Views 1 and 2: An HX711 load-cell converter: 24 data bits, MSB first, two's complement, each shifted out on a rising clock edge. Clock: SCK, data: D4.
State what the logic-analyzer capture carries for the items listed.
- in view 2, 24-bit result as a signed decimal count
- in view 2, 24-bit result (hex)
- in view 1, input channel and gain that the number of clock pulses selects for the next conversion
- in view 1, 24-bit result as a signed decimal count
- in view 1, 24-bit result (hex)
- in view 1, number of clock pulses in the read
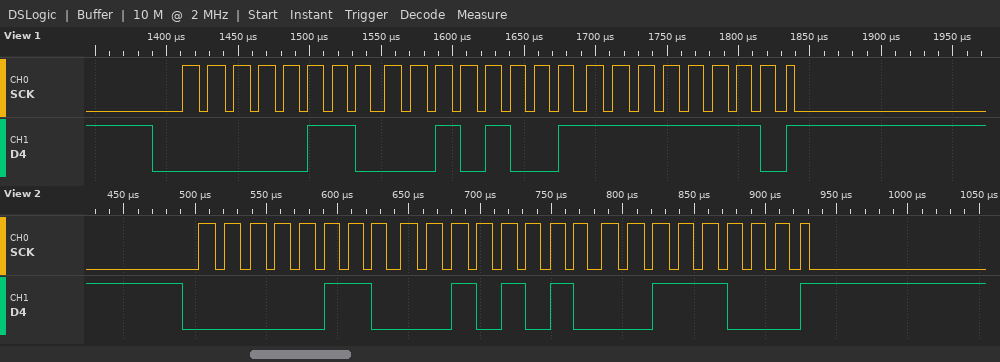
404024
0x062A38
channel A, gain 128
403966
0x0629FE
25
